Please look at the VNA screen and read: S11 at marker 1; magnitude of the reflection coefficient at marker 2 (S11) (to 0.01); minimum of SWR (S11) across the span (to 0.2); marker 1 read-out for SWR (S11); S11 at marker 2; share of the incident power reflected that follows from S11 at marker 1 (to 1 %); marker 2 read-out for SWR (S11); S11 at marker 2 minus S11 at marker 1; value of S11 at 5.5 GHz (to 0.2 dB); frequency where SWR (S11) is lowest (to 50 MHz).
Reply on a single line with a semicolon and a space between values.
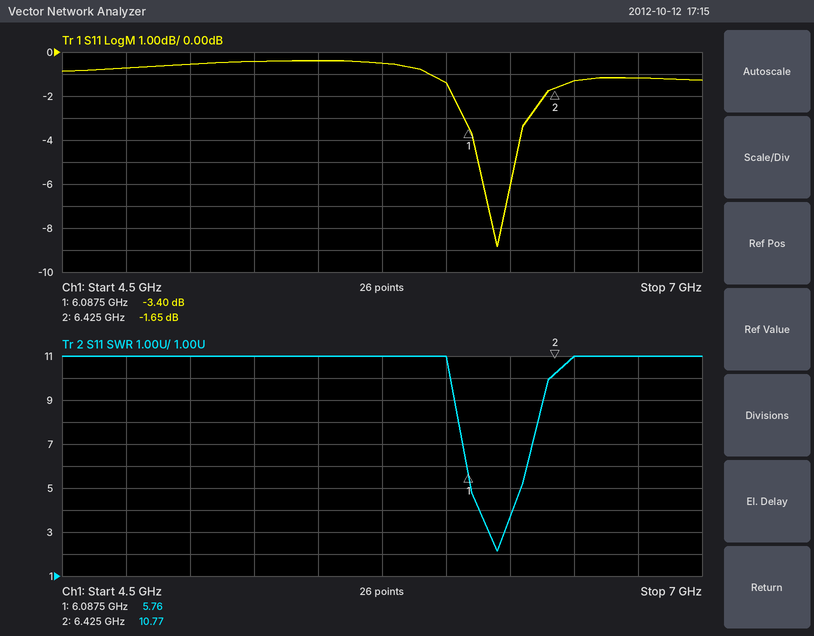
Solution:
-3.40 dB; 0.83; 2.2; 5.76; -1.65 dB; 46 %; 10.77; 1.75 dB; -0.4 dB; 6.20 GHz
